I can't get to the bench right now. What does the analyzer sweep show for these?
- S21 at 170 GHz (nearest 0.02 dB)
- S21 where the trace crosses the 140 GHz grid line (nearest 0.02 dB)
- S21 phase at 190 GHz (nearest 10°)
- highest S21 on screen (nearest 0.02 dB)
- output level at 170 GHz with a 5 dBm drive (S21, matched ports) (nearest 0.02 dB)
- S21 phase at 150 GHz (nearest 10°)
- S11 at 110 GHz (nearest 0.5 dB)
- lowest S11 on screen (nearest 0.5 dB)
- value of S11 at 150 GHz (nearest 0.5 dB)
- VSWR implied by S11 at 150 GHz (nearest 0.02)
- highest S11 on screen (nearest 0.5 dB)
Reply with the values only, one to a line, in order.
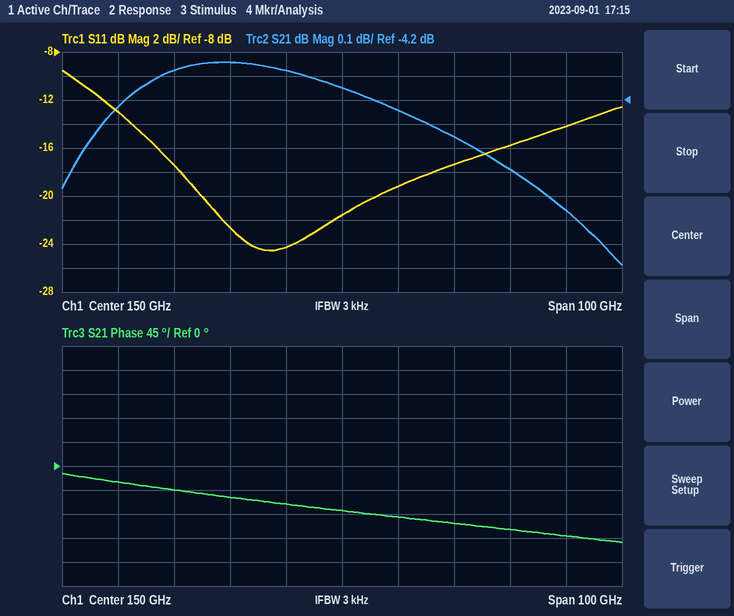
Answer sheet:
-4.36 dB
-4.08 dB
-130°
-4.04 dB
0.64 dBm
-80°
-13.0 dB
-24.5 dB
-21.5 dB
1.18
-9.5 dB
